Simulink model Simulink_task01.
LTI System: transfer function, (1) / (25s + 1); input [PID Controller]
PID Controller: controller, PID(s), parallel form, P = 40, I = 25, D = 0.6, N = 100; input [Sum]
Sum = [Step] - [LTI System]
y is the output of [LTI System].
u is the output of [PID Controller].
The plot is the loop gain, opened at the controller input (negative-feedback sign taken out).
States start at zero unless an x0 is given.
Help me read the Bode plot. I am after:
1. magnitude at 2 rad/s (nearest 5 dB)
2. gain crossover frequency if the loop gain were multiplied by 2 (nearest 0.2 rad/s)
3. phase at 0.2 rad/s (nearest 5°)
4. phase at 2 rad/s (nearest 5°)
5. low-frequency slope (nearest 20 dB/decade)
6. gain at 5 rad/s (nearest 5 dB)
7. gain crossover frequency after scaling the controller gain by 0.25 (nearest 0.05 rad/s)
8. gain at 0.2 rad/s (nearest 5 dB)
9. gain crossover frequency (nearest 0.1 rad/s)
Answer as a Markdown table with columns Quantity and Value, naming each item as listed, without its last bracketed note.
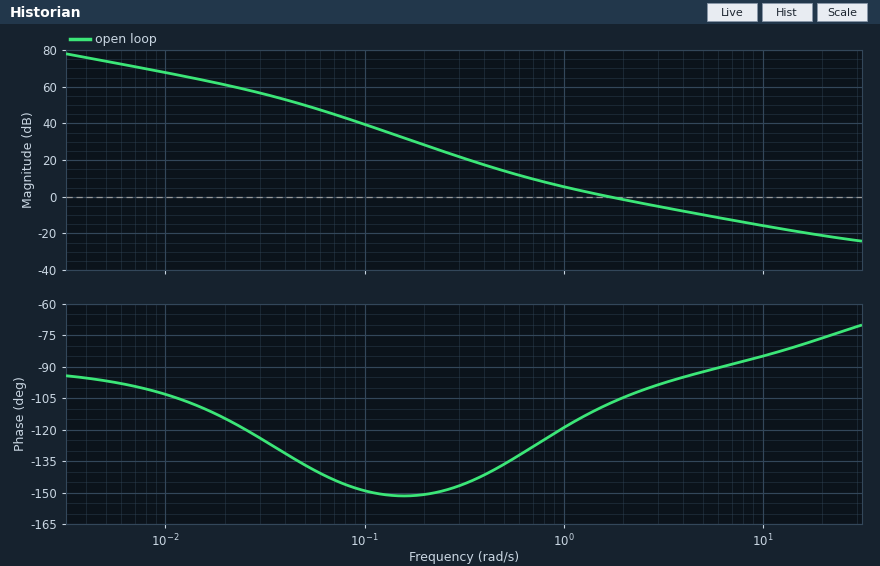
| Quantity | Value |
|---|---|
| magnitude at 2 rad/s | 0 dB |
| gain crossover frequency if the loop gain were multiplied by 2 | 3.2 rad/s |
| phase at 0.2 rad/s | -150° |
| phase at 2 rad/s | -105° |
| low-frequency slope | -20 dB/decade |
| gain at 5 rad/s | -10 dB |
| gain crossover frequency after scaling the controller gain by 0.25 | 0.60 rad/s |
| gain at 0.2 rad/s | 30 dB |
| gain crossover frequency | 1.7 rad/s |
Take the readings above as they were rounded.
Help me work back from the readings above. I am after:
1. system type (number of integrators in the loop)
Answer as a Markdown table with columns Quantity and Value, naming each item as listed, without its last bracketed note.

| Quantity | Value |
|---|---|
| system type | 1 |
